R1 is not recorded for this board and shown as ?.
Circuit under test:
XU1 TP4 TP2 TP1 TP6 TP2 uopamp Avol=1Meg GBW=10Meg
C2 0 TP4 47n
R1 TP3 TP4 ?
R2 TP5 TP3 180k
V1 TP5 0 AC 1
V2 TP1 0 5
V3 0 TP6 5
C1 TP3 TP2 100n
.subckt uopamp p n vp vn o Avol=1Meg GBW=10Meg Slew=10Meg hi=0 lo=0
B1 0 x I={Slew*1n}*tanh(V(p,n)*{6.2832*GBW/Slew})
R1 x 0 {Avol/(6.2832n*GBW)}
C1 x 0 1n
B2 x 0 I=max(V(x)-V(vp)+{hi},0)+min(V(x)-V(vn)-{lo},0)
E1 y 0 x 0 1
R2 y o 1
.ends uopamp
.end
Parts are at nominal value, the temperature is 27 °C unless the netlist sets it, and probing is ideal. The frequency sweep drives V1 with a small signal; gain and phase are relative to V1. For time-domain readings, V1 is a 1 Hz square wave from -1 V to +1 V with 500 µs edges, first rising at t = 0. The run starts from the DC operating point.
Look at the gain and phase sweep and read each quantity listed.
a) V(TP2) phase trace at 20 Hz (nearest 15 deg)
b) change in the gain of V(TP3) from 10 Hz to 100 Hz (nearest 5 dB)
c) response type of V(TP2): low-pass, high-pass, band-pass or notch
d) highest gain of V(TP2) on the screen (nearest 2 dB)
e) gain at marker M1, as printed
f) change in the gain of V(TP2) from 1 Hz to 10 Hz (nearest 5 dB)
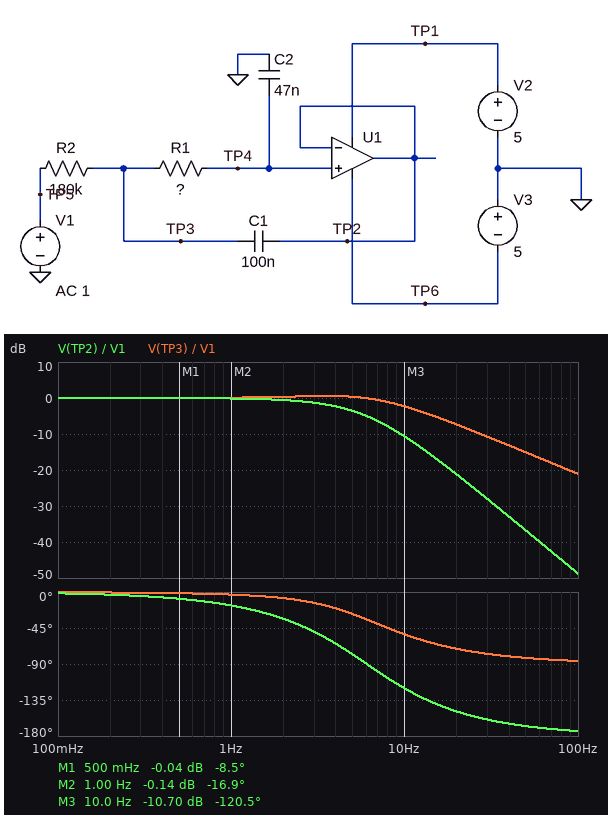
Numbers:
-150 deg
-20 dB
low-pass
0 dB
-0.04 dB
-10 dB
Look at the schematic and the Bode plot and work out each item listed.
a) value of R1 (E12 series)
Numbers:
820 kΩ
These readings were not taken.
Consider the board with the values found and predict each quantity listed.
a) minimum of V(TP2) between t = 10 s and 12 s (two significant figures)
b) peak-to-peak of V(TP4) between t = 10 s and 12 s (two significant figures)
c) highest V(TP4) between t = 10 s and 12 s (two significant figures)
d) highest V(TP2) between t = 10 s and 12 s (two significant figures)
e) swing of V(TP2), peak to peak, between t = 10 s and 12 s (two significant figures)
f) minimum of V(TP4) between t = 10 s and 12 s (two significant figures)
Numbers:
-1.0 V
2.0 V
1.0 V
1.0 V
2.0 V
-1.0 V
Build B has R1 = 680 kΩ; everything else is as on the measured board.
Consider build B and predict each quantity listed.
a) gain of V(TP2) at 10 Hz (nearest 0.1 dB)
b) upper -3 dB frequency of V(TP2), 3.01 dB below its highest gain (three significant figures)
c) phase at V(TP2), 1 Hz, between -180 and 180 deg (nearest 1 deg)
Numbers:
-9.1 dB
5.41 Hz
-15 deg
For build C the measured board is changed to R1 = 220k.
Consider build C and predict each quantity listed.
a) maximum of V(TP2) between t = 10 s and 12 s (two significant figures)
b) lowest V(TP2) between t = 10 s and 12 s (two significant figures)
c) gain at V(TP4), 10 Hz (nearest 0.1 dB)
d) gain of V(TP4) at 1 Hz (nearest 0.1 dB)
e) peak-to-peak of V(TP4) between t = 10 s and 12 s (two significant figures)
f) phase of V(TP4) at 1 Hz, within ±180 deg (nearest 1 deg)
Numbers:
1.1 V
-1.1 V
-1.7 dB
0 dB
2.2 V
-7 deg
